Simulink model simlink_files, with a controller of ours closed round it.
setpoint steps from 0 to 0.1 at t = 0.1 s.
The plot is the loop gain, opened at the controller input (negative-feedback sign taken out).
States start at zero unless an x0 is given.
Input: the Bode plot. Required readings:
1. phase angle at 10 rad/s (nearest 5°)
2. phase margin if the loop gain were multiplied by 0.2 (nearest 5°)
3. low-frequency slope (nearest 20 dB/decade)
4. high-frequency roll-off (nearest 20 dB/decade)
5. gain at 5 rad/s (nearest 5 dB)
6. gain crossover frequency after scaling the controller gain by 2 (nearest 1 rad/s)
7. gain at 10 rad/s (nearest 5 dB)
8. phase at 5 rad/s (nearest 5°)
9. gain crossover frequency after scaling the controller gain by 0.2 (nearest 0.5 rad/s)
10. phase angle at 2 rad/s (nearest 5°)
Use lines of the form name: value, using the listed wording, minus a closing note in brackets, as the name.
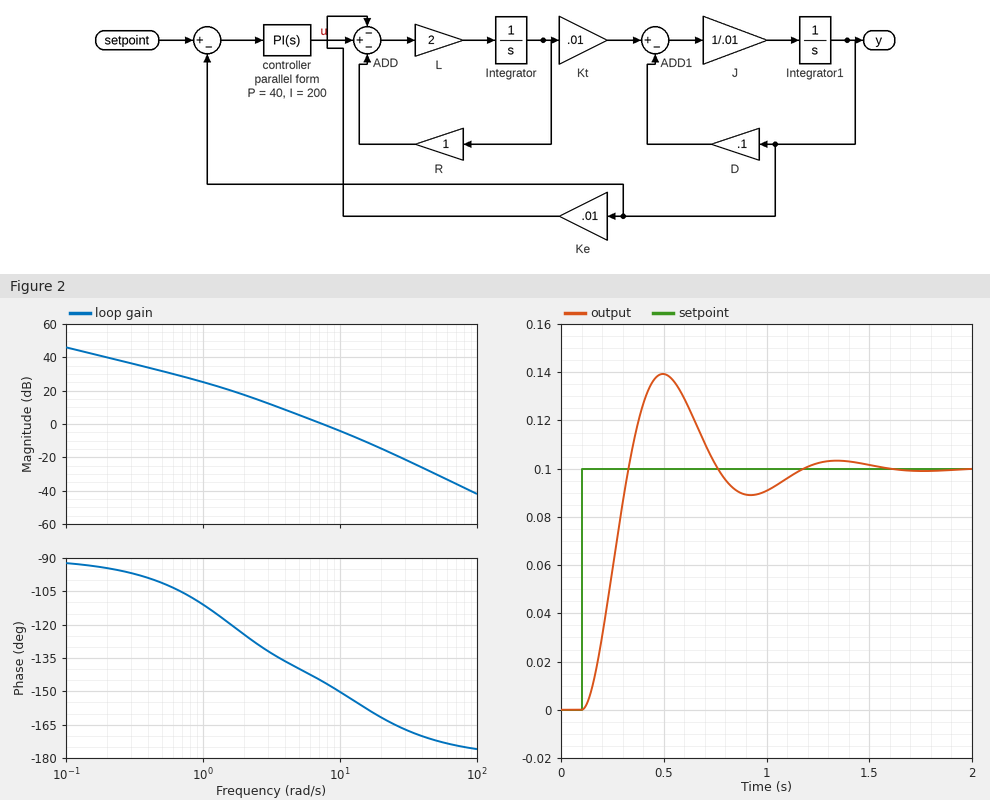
phase angle at 10 rad/s: -150°
phase margin if the loop gain were multiplied by 0.2: 50°
low-frequency slope: -20 dB/decade
high-frequency roll-off: -40 dB/decade
gain at 5 rad/s: 5 dB
gain crossover frequency after scaling the controller gain by 2: 11 rad/s
gain at 10 rad/s: -5 dB
phase at 5 rad/s: -140°
gain crossover frequency after scaling the controller gain by 0.2: 2.5 rad/s
phase angle at 2 rad/s: -125°
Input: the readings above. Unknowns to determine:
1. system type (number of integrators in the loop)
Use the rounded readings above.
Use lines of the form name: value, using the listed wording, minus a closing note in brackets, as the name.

system type: 1
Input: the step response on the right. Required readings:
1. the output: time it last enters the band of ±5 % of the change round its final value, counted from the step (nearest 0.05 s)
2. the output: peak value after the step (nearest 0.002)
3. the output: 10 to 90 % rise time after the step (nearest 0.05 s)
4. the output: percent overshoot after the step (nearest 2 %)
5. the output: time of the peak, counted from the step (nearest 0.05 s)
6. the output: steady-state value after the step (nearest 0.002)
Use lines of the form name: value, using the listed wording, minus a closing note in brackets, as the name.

the output: time it last enters the band of ±5 % of the change round its final value, counted from the step: 1.00 s
the output: peak value after the step: 0.140
the output: 10 to 90 % rise time after the step: 0.15 s
the output: percent overshoot after the step: 40 %
the output: time of the peak, counted from the step: 0.40 s
the output: steady-state value after the step: 0.100
